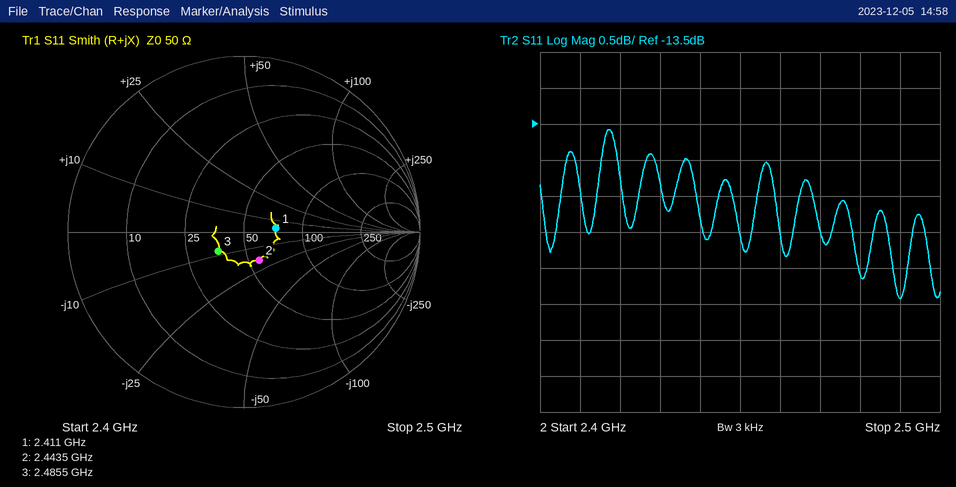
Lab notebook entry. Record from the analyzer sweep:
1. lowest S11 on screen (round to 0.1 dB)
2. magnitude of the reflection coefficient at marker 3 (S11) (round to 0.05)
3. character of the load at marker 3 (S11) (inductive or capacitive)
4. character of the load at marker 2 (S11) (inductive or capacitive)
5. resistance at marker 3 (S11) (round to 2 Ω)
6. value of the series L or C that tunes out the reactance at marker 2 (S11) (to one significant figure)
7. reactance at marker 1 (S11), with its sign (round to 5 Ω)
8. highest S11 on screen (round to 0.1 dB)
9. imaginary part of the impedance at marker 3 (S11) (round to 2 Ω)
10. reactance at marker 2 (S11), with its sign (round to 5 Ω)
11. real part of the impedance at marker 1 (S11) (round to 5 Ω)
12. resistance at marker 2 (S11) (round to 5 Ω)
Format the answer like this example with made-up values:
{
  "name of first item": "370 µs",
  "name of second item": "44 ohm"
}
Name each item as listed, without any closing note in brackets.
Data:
{
  "lowest S11 on screen": "-15.9 dB",
  "magnitude of the reflection coefficient at marker 3 (S11)": "0.20",
  "character of the load at marker 3 (S11)": "capacitive",
  "character of the load at marker 2 (S11)": "capacitive",
  "resistance at marker 3 (S11)": "36 Ω",
  "value of the series L or C that tunes out the reactance at marker 2 (S11)": "1 nH",
  "reactance at marker 1 (S11), with its sign": "+5 Ω",
  "highest S11 on screen": "-13.6 dB",
  "imaginary part of the impedance at marker 3 (S11)": "-8 Ω",
  "reactance at marker 2 (S11), with its sign": "-20 Ω",
  "real part of the impedance at marker 1 (S11)": "70 Ω",
  "resistance at marker 2 (S11)": "55 Ω"
}
